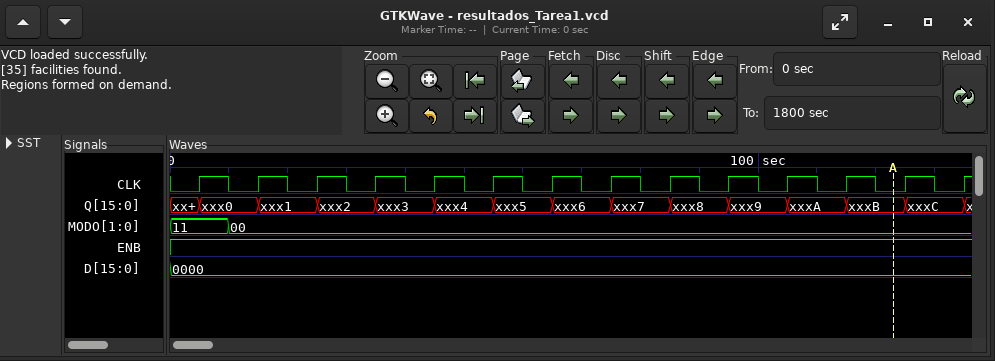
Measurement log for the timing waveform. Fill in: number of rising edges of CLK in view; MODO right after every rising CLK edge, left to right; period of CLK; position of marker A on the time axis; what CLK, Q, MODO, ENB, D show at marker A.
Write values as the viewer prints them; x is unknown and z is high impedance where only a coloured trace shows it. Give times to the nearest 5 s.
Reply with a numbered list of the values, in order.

1. 14
2. 11, 00, 00, 00, 00, 00, 00, 00, 00, 00, 00, 00, 00, 00
3. 10 s
4. 125 s
5. CLK=0, Q=xxxB, MODO=00, ENB=1, D=0000
